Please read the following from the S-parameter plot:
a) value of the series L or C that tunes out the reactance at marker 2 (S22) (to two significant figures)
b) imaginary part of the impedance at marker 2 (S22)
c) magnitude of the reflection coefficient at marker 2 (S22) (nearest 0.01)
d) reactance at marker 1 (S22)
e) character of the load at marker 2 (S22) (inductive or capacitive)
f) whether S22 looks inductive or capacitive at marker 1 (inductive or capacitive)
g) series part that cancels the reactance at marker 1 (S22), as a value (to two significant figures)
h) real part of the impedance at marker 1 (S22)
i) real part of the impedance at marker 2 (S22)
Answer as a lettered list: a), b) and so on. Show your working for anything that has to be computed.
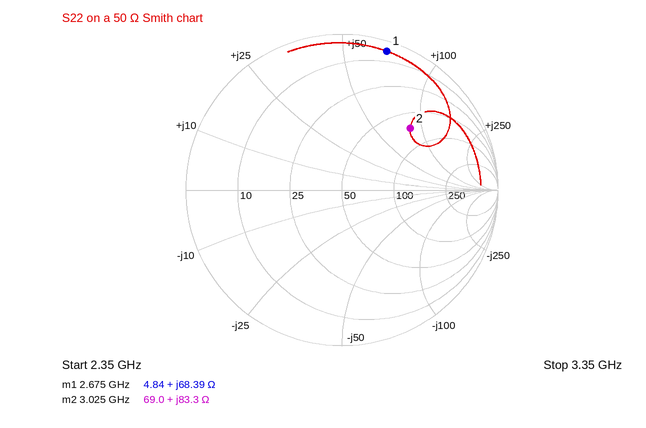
a) C = 1/(2π × 3.025 GHz × 83.3 Ω) ≈ 632 fF, so 630 fF to two significant figures
b) +83.3 Ω
c) 0.59
d) +68.39 Ω
e) inductive
f) inductive
g) C = 1/(2π × 2.675 GHz × 68.39 Ω) ≈ 870 fF
h) 4.84 Ω
i) 69.0 Ω
